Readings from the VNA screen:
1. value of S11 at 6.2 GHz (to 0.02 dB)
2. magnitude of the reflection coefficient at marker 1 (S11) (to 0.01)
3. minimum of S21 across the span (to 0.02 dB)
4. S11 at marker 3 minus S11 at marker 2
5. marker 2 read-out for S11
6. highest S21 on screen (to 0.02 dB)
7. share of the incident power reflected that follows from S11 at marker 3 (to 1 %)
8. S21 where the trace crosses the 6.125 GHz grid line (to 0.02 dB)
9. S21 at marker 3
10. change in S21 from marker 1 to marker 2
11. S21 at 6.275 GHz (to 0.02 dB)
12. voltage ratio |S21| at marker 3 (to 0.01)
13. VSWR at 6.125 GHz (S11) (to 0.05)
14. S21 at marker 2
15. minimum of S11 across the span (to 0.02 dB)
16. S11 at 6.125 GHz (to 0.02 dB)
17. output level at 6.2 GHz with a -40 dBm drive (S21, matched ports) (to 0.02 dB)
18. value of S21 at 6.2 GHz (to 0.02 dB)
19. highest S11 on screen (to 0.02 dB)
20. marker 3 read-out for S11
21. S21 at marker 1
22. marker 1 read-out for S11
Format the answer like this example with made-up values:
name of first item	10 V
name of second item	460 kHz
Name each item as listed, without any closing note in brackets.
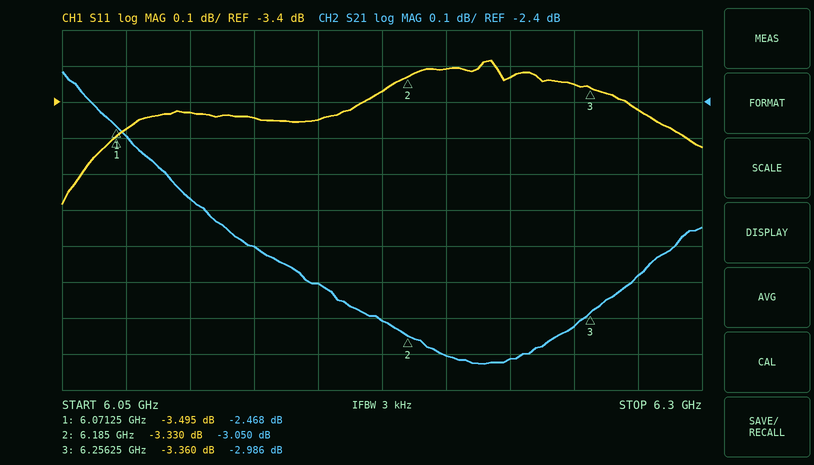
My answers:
value of S11 at 6.2 GHz	-3.30 dB
magnitude of the reflection coefficient at marker 1 (S11)	0.67
minimum of S21 across the span	-3.12 dB
S11 at marker 3 minus S11 at marker 2	-0.030 dB
marker 2 read-out for S11	-3.330 dB
highest S21 on screen	-2.32 dB
share of the incident power reflected that follows from S11 at marker 3	46 %
S21 where the trace crosses the 6.125 GHz grid line	-2.80 dB
S21 at marker 3	-2.986 dB
change in S21 from marker 1 to marker 2	-0.582 dB
S21 at 6.275 GHz	-2.88 dB
voltage ratio |S21| at marker 3	0.71
VSWR at 6.125 GHz (S11)	5.10
S21 at marker 2	-3.050 dB
minimum of S11 across the span	-3.68 dB
S11 at 6.125 GHz	-3.44 dB
output level at 6.2 GHz with a -40 dBm drive (S21, matched ports)	-43.10 dBm
value of S21 at 6.2 GHz	-3.10 dB
highest S11 on screen	-3.28 dB
marker 3 read-out for S11	-3.360 dB
S21 at marker 1	-2.468 dB
marker 1 read-out for S11	-3.495 dB
